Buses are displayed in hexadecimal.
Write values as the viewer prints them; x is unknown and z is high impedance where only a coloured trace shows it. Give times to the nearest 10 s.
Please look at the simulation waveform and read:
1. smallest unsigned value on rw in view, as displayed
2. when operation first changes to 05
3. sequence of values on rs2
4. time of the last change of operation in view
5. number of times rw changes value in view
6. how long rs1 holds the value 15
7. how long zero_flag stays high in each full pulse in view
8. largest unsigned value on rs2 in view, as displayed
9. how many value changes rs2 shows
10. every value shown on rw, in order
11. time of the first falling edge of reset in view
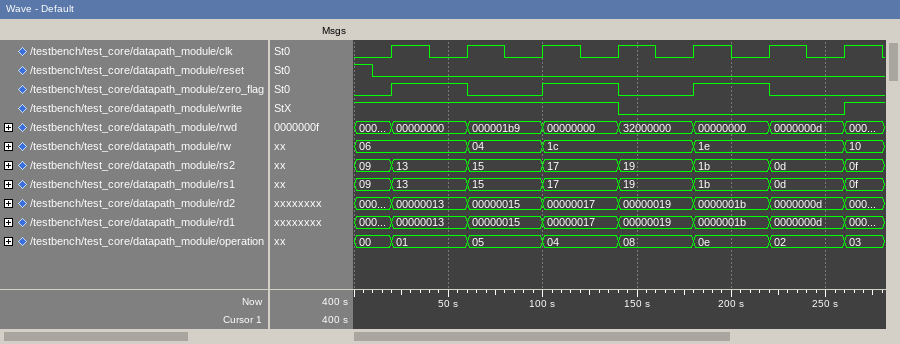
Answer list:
04
60 s
09, 13, 15, 17, 19, 1b, 0d, 0f
260 s
4
40 s
40 s, 40 s, 40 s
1b
7
06, 04, 1c, 1e, 10
10 s
